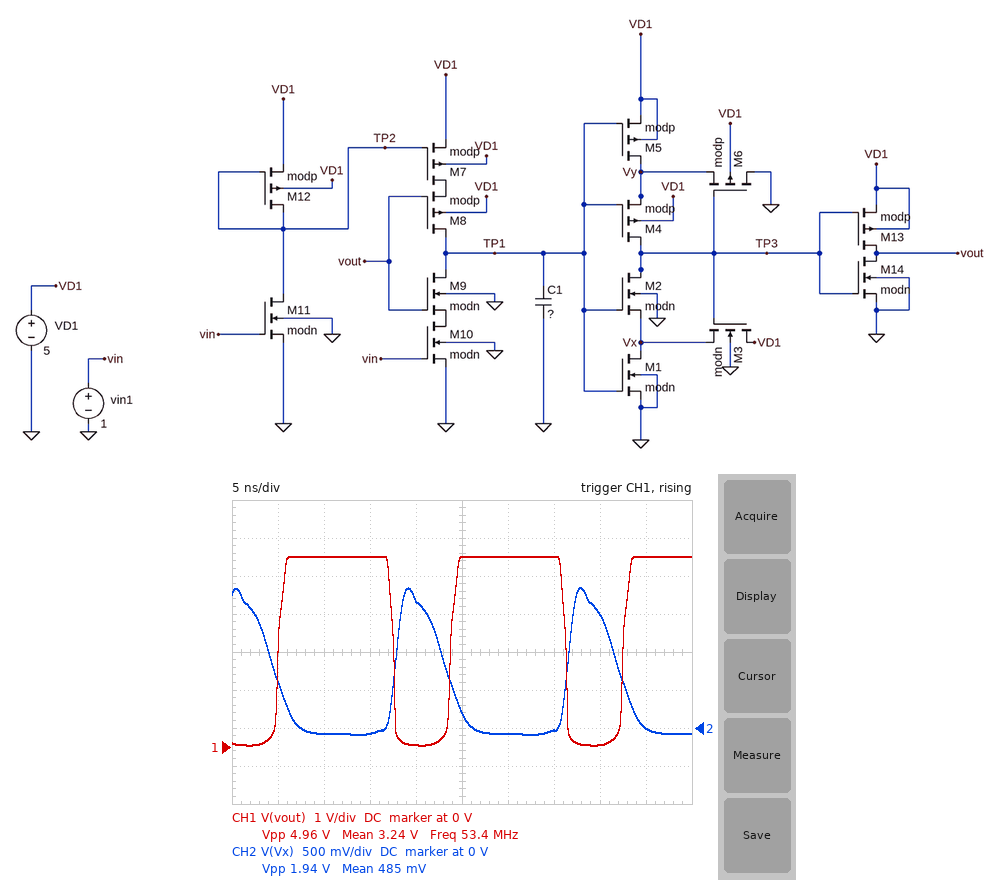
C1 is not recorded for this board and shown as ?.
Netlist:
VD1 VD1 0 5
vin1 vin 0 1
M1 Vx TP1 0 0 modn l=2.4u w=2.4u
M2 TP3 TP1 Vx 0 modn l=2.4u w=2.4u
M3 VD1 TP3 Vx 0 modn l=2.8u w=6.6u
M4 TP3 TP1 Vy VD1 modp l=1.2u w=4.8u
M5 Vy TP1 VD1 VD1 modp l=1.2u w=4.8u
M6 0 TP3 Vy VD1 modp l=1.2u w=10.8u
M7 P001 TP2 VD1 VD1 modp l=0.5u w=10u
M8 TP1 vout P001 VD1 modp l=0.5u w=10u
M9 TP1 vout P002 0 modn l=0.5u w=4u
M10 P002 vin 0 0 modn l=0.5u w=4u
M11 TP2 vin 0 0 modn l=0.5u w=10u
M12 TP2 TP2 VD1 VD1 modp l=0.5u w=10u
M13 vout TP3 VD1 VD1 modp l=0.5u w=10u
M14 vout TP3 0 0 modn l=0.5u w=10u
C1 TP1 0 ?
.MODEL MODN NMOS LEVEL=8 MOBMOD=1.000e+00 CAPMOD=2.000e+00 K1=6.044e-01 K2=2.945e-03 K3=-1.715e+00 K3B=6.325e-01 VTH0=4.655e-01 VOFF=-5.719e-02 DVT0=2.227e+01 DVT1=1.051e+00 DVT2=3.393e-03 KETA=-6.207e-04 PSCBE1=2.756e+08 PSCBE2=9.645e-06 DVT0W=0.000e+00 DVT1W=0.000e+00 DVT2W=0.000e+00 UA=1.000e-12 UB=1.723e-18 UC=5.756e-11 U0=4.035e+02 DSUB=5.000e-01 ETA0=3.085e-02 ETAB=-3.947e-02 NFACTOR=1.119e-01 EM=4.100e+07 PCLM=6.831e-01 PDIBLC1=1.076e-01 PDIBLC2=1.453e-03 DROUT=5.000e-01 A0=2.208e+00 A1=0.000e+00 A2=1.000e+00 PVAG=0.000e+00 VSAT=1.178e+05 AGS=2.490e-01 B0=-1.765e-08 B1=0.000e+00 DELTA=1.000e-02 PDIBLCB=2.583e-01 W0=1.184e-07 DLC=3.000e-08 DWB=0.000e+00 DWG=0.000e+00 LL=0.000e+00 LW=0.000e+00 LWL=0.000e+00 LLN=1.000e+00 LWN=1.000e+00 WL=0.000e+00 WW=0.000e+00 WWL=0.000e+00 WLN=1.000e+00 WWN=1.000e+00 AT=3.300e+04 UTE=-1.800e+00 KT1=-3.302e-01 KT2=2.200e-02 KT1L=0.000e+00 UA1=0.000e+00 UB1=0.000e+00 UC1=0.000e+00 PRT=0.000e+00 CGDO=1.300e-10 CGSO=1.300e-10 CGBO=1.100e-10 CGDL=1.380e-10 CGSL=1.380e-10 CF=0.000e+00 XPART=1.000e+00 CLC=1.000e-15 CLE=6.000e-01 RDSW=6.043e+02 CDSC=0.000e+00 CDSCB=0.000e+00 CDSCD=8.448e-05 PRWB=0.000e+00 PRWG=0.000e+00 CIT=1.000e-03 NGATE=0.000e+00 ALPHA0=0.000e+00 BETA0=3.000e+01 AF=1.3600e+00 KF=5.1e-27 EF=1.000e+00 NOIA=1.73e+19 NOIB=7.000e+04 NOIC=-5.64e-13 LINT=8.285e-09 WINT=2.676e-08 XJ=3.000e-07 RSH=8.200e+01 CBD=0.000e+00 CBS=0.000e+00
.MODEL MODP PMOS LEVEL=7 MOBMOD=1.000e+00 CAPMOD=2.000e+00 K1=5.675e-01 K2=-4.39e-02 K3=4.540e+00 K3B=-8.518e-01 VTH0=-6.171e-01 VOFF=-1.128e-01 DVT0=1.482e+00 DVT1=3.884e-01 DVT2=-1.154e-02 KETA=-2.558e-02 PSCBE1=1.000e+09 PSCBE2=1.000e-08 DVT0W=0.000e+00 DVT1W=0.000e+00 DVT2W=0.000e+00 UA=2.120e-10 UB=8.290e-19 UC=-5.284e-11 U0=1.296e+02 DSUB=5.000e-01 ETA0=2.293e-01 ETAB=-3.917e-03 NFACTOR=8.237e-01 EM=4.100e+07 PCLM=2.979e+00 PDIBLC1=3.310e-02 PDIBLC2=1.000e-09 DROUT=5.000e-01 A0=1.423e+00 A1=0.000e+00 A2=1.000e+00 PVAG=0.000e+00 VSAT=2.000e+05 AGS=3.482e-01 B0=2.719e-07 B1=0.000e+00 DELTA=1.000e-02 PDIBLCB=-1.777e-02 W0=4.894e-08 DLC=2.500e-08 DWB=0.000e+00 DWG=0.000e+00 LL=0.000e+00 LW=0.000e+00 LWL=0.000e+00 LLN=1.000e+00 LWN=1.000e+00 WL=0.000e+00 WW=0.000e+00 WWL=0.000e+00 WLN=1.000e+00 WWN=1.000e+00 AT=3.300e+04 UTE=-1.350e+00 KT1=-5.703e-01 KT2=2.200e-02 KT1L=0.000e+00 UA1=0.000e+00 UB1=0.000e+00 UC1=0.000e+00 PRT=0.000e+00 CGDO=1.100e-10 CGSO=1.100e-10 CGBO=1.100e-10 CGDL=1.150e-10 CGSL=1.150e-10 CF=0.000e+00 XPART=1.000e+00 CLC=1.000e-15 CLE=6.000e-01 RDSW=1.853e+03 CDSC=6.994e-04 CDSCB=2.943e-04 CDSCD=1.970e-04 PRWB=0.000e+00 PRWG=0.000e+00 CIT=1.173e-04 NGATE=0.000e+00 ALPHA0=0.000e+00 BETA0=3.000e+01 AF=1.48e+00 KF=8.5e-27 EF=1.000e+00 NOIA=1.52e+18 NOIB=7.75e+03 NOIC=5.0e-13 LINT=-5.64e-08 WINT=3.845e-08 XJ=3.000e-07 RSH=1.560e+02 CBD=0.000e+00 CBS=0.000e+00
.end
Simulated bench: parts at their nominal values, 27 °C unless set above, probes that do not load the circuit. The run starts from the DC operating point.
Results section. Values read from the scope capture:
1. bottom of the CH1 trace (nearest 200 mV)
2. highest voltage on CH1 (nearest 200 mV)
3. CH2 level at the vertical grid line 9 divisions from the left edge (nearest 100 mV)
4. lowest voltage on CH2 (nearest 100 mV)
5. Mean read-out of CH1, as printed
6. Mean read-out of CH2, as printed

0 V
5.0 V
0 V
-100 mV
3.24 V
485 mV
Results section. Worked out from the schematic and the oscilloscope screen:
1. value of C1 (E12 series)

470 fF
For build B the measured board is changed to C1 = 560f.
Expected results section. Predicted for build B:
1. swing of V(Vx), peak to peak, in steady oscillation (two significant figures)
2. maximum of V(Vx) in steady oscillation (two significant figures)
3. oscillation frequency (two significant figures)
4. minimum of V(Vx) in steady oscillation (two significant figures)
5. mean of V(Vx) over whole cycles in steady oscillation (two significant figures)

2.0 V
1.9 V
47 MHz
-79 mV
490 mV
